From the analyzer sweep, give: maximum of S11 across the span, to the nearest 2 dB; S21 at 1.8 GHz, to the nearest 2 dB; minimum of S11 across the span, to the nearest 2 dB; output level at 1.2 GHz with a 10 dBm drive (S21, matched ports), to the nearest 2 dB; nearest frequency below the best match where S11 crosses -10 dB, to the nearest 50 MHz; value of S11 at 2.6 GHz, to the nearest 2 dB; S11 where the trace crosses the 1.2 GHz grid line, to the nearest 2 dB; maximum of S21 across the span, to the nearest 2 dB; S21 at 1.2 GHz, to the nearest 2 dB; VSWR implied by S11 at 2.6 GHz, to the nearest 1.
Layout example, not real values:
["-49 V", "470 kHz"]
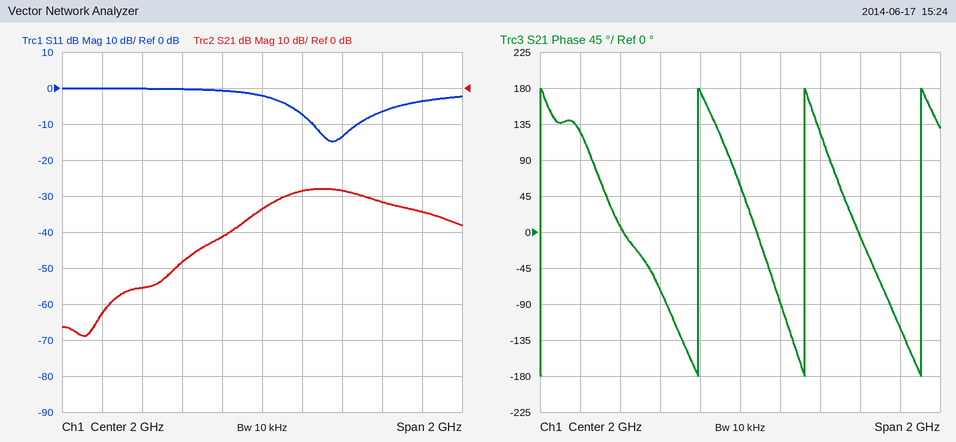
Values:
["0 dB", "-42 dB", "-14 dB", "-52 dBm", "2.25 GHz", "-6 dB", "0 dB", "-28 dB", "-62 dB", "3"]
